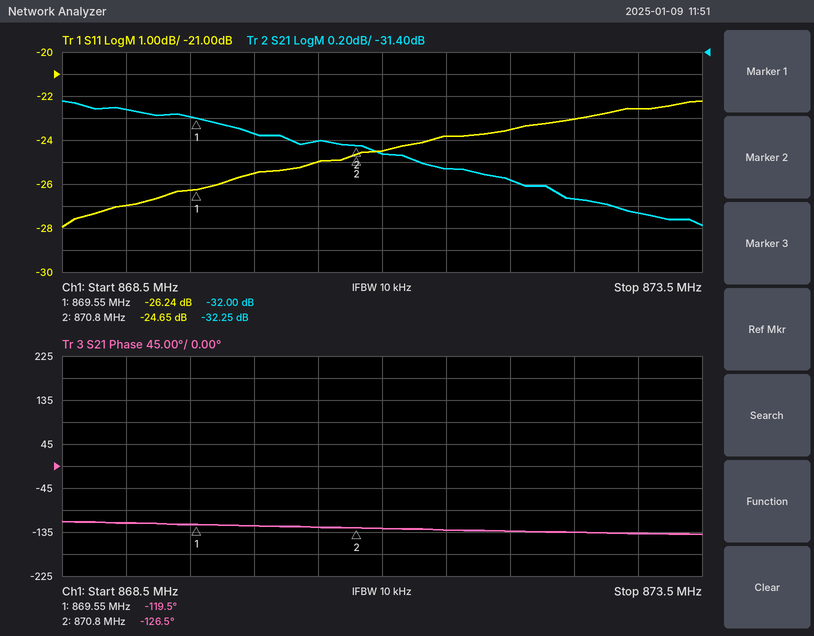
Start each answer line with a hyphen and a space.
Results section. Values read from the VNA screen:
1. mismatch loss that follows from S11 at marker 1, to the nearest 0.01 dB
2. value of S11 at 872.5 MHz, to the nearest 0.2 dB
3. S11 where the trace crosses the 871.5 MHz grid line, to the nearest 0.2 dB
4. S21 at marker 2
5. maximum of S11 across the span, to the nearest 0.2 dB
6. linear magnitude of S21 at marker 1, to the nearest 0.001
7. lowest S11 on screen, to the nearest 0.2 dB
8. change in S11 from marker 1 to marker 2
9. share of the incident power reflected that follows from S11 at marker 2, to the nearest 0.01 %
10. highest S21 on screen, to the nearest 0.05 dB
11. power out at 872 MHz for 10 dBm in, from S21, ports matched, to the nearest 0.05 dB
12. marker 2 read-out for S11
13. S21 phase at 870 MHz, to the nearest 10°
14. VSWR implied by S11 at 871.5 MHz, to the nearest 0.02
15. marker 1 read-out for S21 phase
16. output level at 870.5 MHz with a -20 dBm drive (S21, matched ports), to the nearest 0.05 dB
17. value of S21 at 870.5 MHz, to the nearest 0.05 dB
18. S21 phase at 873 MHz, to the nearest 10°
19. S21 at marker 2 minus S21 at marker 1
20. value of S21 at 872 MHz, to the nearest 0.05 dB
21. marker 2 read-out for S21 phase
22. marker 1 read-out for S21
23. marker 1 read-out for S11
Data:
- 0.01 dB
- -23.0 dB
- -23.8 dB
- -32.25 dB
- -22.2 dB
- 0.025
- -28.0 dB
- 1.59 dB
- 0.34 %
- -31.85 dB
- -22.55 dBm
- -24.65 dB
- -120°
- 1.14
- -119.5°
- -52.20 dBm
- -32.20 dB
- -140°
- -0.25 dB
- -32.55 dB
- -126.5°
- -32.00 dB
- -26.24 dB
